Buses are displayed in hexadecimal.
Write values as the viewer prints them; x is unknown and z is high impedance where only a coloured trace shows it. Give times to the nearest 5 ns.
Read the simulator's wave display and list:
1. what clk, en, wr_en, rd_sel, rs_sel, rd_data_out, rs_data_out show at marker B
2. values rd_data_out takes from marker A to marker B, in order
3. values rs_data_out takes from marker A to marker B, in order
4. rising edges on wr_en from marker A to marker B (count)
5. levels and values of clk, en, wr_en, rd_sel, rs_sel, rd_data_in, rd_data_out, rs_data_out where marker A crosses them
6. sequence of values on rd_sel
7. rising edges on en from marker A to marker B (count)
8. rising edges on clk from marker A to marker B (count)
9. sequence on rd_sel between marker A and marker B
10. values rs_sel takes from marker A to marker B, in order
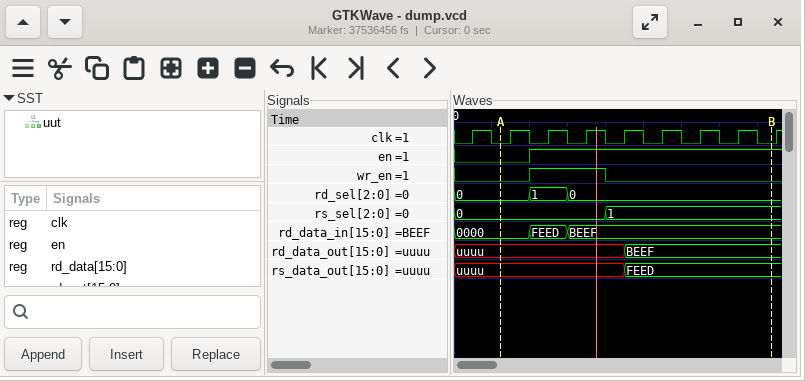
clk=0, en=1, wr_en=0, rd_sel=0, rs_sel=1, rd_data_out=BEEF, rs_data_out=FEED
uuuu, BEEF
uuuu, FEED
1
clk=0, en=0, wr_en=0, rd_sel=0, rs_sel=0, rd_data_in=0000, rd_data_out=uuuu, rs_data_out=uuuu
0, 1, 0
1
7
0, 1, 0
0, 1
